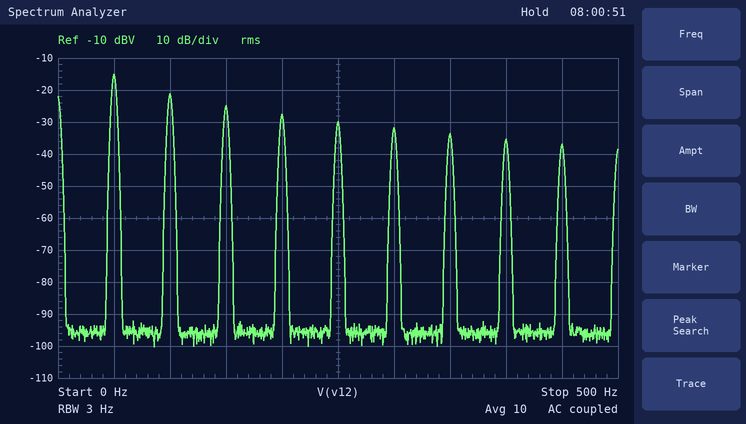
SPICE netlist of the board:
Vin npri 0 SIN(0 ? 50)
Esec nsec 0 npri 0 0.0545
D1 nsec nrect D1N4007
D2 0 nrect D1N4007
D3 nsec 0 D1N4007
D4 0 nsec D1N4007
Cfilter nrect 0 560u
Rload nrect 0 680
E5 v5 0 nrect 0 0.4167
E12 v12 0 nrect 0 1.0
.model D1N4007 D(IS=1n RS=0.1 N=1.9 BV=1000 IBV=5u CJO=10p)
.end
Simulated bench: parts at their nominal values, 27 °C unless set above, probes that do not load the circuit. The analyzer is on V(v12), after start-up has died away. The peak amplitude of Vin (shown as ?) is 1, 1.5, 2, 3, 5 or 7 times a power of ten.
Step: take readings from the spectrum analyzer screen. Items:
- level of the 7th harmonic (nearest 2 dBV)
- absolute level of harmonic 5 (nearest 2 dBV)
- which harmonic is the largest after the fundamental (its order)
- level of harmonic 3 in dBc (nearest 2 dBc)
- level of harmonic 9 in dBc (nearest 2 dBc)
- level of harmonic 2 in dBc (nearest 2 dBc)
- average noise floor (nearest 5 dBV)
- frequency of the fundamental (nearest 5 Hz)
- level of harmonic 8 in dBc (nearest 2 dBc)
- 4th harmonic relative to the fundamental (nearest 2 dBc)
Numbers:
-34 dBV
-30 dBV
2
-10 dBc
-22 dBc
-6 dBc
-95 dBV
50 Hz
-20 dBc
-12 dBc
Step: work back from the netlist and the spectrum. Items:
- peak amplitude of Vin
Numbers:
300 V
